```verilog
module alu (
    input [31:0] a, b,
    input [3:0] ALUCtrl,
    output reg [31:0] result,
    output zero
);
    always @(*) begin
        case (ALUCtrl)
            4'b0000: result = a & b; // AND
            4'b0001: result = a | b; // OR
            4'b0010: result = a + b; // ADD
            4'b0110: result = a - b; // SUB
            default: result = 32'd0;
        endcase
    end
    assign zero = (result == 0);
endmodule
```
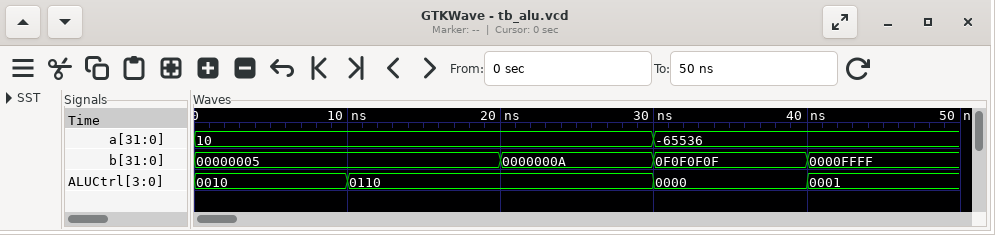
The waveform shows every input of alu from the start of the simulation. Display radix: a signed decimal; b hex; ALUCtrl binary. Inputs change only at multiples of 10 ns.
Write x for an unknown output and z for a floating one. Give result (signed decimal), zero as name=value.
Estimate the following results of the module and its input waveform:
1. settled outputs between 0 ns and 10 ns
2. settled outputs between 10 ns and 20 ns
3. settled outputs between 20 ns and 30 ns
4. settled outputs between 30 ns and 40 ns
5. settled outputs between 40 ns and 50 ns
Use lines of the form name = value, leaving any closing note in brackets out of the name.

settled outputs between 0 ns and 10 ns = result=15, zero=0
settled outputs between 10 ns and 20 ns = result=5, zero=0
settled outputs between 20 ns and 30 ns = result=0, zero=1
settled outputs between 30 ns and 40 ns = result=252641280, zero=0
settled outputs between 40 ns and 50 ns = result=-1, zero=0
